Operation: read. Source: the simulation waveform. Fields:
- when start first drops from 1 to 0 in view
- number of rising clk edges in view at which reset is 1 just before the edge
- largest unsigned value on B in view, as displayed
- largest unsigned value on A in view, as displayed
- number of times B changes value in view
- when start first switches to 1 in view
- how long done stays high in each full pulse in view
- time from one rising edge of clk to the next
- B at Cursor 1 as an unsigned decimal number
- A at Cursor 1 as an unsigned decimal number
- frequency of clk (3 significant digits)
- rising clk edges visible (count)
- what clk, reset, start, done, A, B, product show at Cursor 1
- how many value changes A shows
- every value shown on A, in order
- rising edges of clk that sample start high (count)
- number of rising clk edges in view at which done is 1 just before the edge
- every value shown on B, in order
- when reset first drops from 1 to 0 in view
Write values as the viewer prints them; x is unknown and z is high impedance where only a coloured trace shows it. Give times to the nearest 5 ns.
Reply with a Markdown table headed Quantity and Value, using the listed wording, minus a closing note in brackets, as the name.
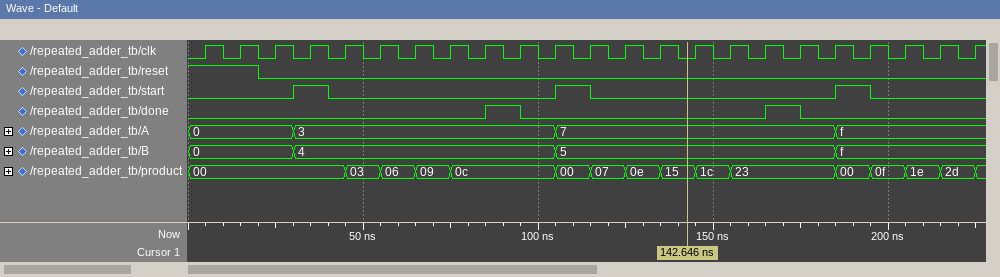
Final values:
| Quantity | Value |
|---|---|
| when start first drops from 1 to 0 in view | 40 ns |
| number of rising clk edges in view at which reset is 1 just before the edge | 2 |
| largest unsigned value on B in view, as displayed | f |
| largest unsigned value on A in view, as displayed | f |
| number of times B changes value in view | 3 |
| when start first switches to 1 in view | 30 ns |
| how long done stays high in each full pulse in view | 10 ns, 10 ns |
| time from one rising edge of clk to the next | 10 ns |
| B at Cursor 1 as an unsigned decimal number | 5 |
| A at Cursor 1 as an unsigned decimal number | 7 |
| frequency of clk | 100 MHz |
| rising clk edges visible | 23 |
| what clk, reset, start, done, A, B, product show at Cursor 1 | clk=0, reset=0, start=0, done=0, A=7, B=5, product=15 |
| how many value changes A shows | 3 |
| every value shown on A, in order | 0, 3, 7, f |
| rising edges of clk that sample start high | 3 |
| number of rising clk edges in view at which done is 1 just before the edge | 2 |
| every value shown on B, in order | 0, 4, 5, f |
| when reset first drops from 1 to 0 in view | 20 ns |
